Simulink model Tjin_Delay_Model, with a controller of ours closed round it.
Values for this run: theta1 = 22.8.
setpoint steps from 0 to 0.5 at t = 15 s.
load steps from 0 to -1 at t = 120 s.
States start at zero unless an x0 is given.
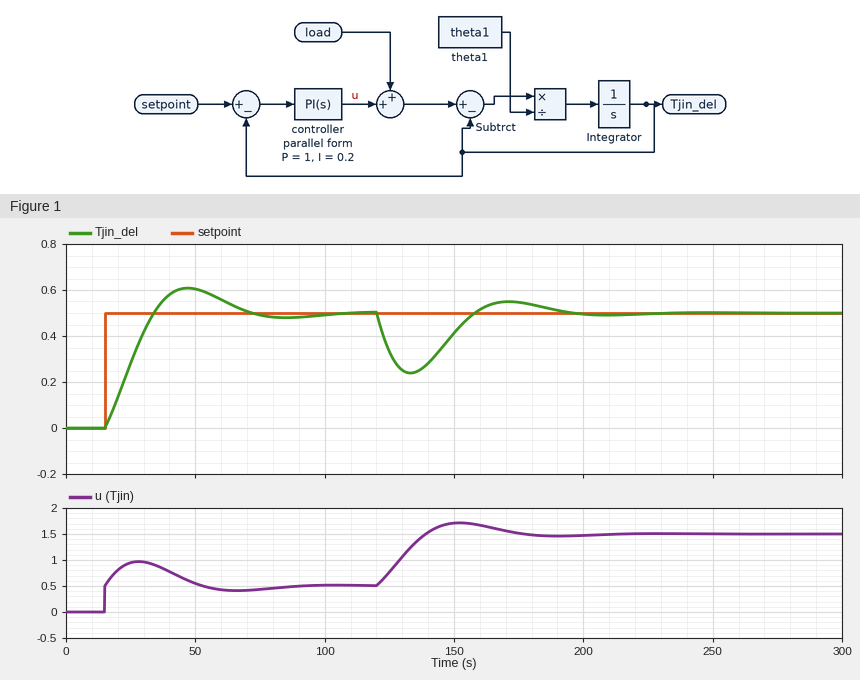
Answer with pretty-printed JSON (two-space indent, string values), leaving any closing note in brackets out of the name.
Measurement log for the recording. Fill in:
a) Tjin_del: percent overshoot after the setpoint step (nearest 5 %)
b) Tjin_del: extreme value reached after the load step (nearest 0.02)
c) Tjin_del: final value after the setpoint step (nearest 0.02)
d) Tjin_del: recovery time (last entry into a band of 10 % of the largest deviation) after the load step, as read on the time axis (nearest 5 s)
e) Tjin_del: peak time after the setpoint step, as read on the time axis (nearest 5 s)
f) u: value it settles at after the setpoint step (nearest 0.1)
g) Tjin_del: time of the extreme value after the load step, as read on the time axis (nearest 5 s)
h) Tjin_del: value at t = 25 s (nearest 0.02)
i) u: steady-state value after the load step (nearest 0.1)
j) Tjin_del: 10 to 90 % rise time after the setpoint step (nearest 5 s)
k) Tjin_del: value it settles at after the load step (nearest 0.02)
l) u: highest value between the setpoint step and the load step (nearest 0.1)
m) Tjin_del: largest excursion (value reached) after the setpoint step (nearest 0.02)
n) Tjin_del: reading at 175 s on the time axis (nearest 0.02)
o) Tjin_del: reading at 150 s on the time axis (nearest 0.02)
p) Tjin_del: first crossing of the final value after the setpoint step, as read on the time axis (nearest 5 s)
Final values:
{
  "Tjin_del: percent overshoot after the setpoint step": "20 %",
  "Tjin_del: extreme value reached after the load step": "0.24",
  "Tjin_del: final value after the setpoint step": "0.50",
  "Tjin_del: recovery time (last entry into a band of 10 % of the largest deviation) after the load step, as read on the time axis": "185 s",
  "Tjin_del: peak time after the setpoint step, as read on the time axis": "45 s",
  "u: value it settles at after the setpoint step": "0.5",
  "Tjin_del: time of the extreme value after the load step, as read on the time axis": "135 s",
  "Tjin_del: value at t = 25 s": "0.28",
  "u: steady-state value after the load step": "1.5",
  "Tjin_del: 10 to 90 % rise time after the setpoint step": "15 s",
  "Tjin_del: value it settles at after the load step": "0.50",
  "u: highest value between the setpoint step and the load step": "1.0",
  "Tjin_del: largest excursion (value reached) after the setpoint step": "0.60",
  "Tjin_del: reading at 175 s on the time axis": "0.54",
  "Tjin_del: reading at 150 s on the time axis": "0.42",
  "Tjin_del: first crossing of the final value after the setpoint step, as read on the time axis": "35 s"
}
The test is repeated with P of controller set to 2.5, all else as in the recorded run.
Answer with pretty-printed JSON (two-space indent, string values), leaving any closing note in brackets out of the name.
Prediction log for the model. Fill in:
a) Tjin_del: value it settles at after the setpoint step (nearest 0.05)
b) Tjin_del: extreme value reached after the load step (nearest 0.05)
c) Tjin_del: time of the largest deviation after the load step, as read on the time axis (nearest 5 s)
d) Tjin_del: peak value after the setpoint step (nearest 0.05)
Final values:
{
  "Tjin_del: value it settles at after the setpoint step": "0.50",
  "Tjin_del: extreme value reached after the load step": "0.30",
  "Tjin_del: time of the largest deviation after the load step, as read on the time axis": "130 s",
  "Tjin_del: peak value after the setpoint step": "0.55"
}
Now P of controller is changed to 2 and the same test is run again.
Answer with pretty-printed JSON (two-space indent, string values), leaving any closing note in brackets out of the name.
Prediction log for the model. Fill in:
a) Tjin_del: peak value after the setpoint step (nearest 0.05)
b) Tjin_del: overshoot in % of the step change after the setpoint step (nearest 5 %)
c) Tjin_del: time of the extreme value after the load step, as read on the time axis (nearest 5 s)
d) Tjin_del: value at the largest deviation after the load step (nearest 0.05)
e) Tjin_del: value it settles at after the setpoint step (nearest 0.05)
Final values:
{
  "Tjin_del: peak value after the setpoint step": "0.55",
  "Tjin_del: overshoot in % of the step change after the setpoint step": "10 %",
  "Tjin_del: time of the extreme value after the load step, as read on the time axis": "130 s",
  "Tjin_del: value at the largest deviation after the load step": "0.30",
  "Tjin_del: value it settles at after the setpoint step": "0.50"
}
